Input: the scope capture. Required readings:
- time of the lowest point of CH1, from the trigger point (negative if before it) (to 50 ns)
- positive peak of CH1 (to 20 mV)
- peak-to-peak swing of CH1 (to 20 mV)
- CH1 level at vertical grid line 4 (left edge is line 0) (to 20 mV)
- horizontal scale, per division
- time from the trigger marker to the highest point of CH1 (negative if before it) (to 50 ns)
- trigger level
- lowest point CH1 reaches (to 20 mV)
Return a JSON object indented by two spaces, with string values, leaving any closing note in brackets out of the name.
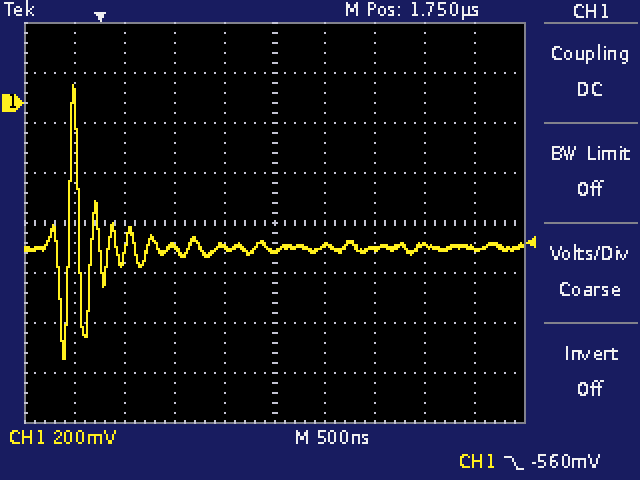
{
  "time of the lowest point of CH1, from the trigger point (negative if before it)": "-350 ns",
  "positive peak of CH1": "80 mV",
  "peak-to-peak swing of CH1": "1.10 V",
  "CH1 level at vertical grid line 4 (left edge is line 0)": "-580 mV",
  "horizontal scale, per division": "500 ns",
  "time from the trigger marker to the highest point of CH1 (negative if before it)": "-250 ns",
  "trigger level": "-560 mV",
  "lowest point CH1 reaches": "-1.02 V"
}
